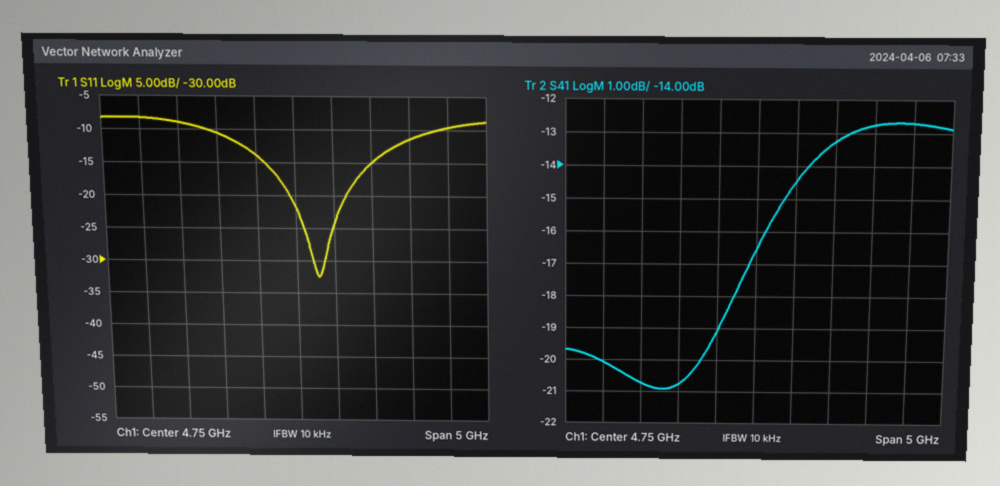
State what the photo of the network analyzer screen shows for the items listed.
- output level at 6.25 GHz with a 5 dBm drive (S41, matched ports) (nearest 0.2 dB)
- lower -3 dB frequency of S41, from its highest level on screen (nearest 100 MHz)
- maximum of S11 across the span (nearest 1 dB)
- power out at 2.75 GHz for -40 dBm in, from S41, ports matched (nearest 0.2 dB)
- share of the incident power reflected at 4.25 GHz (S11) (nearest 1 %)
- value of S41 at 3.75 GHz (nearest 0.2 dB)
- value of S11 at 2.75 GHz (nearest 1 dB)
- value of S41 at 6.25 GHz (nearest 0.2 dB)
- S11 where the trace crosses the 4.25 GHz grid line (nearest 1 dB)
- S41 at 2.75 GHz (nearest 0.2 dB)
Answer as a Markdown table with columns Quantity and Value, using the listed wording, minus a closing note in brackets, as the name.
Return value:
| Quantity | Value |
|---|---|
| output level at 6.25 GHz with a 5 dBm drive (S41, matched ports) | -7.8 dBm |
| lower -3 dB frequency of S41, from its highest level on screen | 4.9 GHz |
| maximum of S11 across the span | -8 dB |
| power out at 2.75 GHz for -40 dBm in, from S41, ports matched | -60.0 dBm |
| share of the incident power reflected at 4.25 GHz (S11) | 4 % |
| value of S41 at 3.75 GHz | -20.8 dB |
| value of S11 at 2.75 GHz | -8 dB |
| value of S41 at 6.25 GHz | -12.8 dB |
| S11 where the trace crosses the 4.25 GHz grid line | -14 dB |
| S41 at 2.75 GHz | -20.0 dB |
